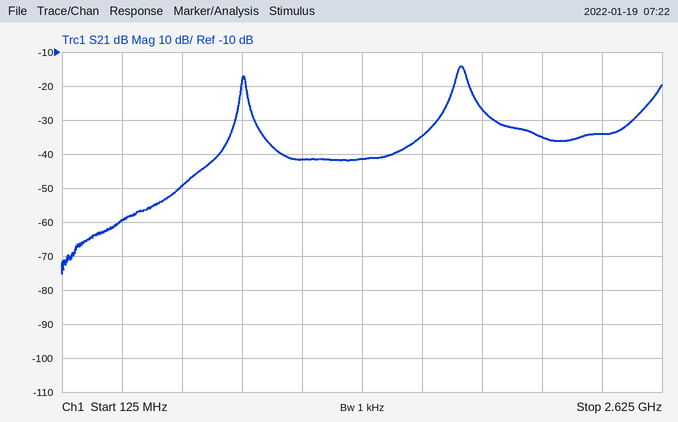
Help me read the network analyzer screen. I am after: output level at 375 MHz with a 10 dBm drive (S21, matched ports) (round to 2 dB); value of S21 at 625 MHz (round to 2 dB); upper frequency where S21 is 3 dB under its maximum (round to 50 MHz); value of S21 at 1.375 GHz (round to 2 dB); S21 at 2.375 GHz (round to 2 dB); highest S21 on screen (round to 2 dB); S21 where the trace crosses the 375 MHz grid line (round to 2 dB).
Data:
-50 dBm
-50 dB
1.80 GHz
-42 dB
-34 dB
-14 dB
-60 dB
